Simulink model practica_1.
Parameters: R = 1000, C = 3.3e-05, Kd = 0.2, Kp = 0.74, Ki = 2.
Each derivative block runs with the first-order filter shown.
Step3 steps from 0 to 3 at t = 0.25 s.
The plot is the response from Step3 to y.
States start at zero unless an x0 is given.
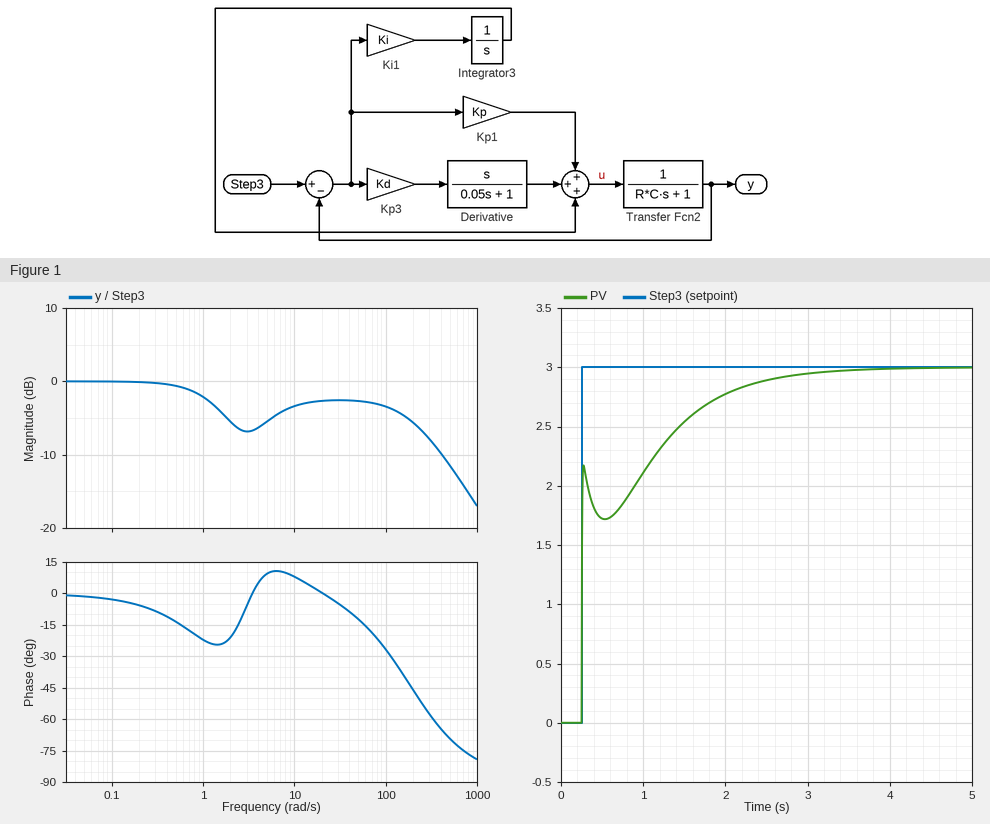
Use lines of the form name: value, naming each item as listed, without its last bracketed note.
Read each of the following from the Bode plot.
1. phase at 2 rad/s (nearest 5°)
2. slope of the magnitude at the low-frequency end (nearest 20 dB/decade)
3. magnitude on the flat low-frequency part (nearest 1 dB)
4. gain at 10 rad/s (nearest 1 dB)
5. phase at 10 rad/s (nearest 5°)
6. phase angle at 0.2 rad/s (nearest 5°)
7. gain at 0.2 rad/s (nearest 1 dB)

phase at 2 rad/s: -20°
slope of the magnitude at the low-frequency end: 0 dB/decade
magnitude on the flat low-frequency part: 0 dB
gain at 10 rad/s: -3 dB
phase at 10 rad/s: 10°
phase angle at 0.2 rad/s: -5°
gain at 0.2 rad/s: 0 dB
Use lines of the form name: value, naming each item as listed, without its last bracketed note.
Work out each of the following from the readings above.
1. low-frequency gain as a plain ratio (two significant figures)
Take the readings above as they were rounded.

low-frequency gain as a plain ratio: 1.0
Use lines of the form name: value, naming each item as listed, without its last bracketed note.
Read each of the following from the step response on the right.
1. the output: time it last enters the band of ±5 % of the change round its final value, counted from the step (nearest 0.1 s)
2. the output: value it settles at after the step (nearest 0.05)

the output: time it last enters the band of ±5 % of the change round its final value, counted from the step: 2.0 s
the output: value it settles at after the step: 3.00
